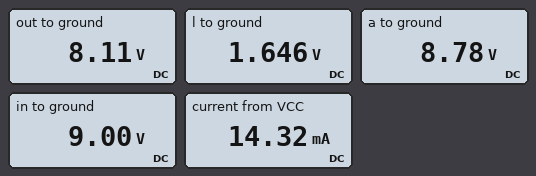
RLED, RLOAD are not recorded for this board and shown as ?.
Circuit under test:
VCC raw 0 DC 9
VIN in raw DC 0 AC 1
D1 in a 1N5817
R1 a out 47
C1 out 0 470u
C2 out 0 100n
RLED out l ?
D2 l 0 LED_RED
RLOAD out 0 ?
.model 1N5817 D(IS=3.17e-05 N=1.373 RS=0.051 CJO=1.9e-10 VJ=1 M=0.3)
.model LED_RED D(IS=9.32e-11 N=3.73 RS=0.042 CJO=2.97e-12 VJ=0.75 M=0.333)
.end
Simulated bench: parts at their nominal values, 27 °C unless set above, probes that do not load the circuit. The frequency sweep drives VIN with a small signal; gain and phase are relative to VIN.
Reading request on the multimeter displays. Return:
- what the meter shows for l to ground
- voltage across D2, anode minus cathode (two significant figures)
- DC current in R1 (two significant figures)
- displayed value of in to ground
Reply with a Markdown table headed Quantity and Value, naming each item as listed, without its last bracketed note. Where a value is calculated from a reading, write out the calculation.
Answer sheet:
| Quantity | Value |
|---|---|
| what the meter shows for l to ground | 1.646 V |
| voltage across D2, anode minus cathode | 1.646 V = 1.6 V |
| DC current in R1 | (8.78 V - 8.11 V) / 47 Ω = 14 mA |
| displayed value of in to ground | 9.00 V |
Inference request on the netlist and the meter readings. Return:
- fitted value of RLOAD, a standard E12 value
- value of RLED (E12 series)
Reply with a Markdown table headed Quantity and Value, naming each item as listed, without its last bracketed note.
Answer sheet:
| Quantity | Value |
|---|---|
| fitted value of RLOAD, a standard E12 value | 680 Ω |
| value of RLED | 2.7 kΩ |
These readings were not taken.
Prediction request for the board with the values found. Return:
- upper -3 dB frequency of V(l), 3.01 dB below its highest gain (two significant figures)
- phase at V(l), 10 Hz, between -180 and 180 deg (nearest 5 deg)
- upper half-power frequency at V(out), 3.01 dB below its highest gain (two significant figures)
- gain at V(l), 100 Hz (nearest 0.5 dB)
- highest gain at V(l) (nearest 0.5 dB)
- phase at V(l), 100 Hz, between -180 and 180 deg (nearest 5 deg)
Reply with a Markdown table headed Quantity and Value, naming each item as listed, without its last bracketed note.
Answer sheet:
| Quantity | Value |
|---|---|
| upper -3 dB frequency of V(l), 3.01 dB below its highest gain | 7.5 Hz |
| phase at V(l), 10 Hz, between -180 and 180 deg | -55 deg |
| upper half-power frequency at V(out), 3.01 dB below its highest gain | 7.5 Hz |
| gain at V(l), 100 Hz | -60.0 dB |
| highest gain at V(l) | -37.5 dB |
| phase at V(l), 100 Hz, between -180 and 180 deg | -85 deg |
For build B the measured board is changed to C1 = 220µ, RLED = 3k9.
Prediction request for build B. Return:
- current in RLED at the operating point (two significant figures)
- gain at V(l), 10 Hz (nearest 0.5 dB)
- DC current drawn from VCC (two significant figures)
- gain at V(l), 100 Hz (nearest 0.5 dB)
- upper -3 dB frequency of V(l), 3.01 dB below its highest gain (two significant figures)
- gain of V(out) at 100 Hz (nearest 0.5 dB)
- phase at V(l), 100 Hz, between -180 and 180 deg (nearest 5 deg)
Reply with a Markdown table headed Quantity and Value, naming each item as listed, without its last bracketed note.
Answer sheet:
| Quantity | Value |
|---|---|
| current in RLED at the operating point | 1.7 mA |
| gain at V(l), 10 Hz | -39.0 dB |
| DC current drawn from VCC | 14 mA |
| gain at V(l), 100 Hz | -53.5 dB |
| upper -3 dB frequency of V(l), 3.01 dB below its highest gain | 16 Hz |
| gain of V(out) at 100 Hz | -17.0 dB |
| phase at V(l), 100 Hz, between -180 and 180 deg | -80 deg |
